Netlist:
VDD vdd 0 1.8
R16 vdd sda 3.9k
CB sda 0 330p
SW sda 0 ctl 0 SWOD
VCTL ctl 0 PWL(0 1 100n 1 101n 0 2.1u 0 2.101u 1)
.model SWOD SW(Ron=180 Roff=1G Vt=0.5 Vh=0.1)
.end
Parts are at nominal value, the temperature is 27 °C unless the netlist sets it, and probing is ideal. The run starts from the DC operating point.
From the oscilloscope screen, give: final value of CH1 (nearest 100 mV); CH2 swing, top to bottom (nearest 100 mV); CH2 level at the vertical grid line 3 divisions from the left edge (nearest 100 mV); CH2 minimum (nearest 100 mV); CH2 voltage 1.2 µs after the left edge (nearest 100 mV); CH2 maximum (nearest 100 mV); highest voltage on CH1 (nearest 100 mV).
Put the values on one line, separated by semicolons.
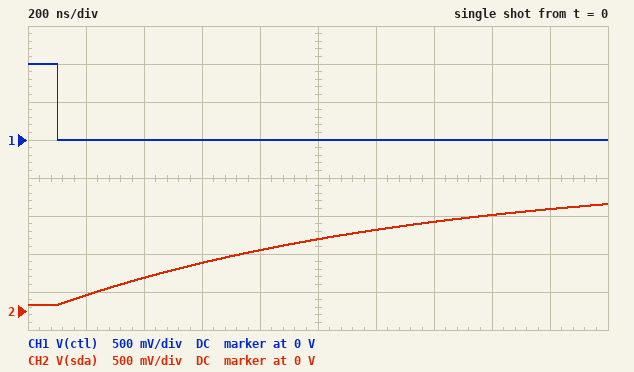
0 V; 1.3 V; 600 mV; 100 mV; 1.1 V; 1.4 V; 1.0 V
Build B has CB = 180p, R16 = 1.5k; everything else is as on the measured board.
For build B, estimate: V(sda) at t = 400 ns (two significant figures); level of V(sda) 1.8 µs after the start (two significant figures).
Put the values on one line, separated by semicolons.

1.3 V; 1.8 V
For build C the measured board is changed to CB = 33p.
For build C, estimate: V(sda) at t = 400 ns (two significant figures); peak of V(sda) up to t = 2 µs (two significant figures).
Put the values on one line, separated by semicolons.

1.6 V; 1.8 V
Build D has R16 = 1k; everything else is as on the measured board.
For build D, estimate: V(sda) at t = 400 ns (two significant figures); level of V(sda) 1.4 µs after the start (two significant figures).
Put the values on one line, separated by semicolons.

1.2 V; 1.8 V
